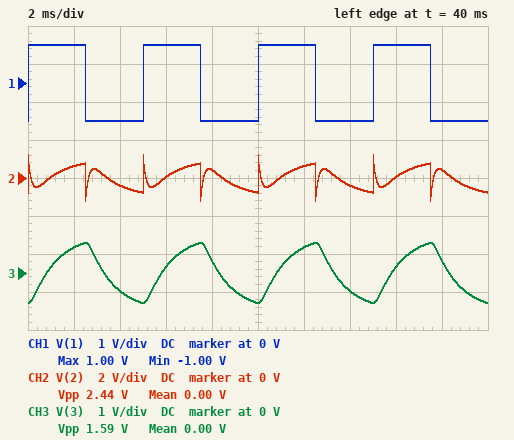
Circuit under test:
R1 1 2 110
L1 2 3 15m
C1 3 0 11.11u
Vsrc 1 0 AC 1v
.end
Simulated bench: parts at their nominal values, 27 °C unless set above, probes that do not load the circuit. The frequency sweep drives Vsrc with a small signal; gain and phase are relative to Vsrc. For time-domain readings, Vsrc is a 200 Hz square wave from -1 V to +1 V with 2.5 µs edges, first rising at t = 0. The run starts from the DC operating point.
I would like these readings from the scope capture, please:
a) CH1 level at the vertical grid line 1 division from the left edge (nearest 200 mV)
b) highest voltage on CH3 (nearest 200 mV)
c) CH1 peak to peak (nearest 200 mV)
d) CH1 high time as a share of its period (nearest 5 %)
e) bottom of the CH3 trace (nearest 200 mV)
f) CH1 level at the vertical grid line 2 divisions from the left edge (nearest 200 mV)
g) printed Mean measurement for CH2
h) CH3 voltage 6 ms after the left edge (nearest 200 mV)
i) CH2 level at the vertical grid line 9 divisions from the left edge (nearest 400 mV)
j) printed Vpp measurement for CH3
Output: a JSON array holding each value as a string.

["1.0 V", "800 mV", "2.0 V", "50 %", "-800 mV", "-1.0 V", "0.00 V", "200 mV", "400 mV", "1.59 V"]
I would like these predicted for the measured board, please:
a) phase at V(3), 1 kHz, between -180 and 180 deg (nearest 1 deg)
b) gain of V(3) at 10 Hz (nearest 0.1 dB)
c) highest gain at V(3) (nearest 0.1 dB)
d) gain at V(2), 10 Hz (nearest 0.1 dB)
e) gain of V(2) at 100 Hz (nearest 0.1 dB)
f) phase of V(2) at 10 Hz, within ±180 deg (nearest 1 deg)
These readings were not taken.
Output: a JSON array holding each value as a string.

["-126 deg", "0 dB", "0 dB", "0 dB", "-2.2 dB", "-4 deg"]
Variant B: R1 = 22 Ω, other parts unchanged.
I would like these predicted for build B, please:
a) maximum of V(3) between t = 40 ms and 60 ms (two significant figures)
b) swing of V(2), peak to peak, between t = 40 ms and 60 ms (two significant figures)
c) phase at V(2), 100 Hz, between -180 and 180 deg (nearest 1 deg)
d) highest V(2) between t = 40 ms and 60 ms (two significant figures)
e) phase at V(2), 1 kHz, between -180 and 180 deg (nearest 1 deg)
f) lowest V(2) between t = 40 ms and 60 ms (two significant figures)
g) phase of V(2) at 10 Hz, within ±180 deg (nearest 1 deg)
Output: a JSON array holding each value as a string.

["1.7 V", "2.5 V", "-9 deg", "1.3 V", "15 deg", "-1.3 V", "-1 deg"]
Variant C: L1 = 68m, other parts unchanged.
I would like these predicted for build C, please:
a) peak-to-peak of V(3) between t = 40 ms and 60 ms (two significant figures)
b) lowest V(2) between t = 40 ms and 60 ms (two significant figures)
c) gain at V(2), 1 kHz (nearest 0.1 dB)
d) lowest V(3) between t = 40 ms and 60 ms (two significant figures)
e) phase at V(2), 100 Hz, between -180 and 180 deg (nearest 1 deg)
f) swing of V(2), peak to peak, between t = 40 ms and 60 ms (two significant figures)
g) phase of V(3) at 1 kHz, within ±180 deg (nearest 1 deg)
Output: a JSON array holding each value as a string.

["1.7 V", "-1.5 V", "-0.3 dB", "-870 mV", "-48 deg", "3.0 V", "-165 deg"]
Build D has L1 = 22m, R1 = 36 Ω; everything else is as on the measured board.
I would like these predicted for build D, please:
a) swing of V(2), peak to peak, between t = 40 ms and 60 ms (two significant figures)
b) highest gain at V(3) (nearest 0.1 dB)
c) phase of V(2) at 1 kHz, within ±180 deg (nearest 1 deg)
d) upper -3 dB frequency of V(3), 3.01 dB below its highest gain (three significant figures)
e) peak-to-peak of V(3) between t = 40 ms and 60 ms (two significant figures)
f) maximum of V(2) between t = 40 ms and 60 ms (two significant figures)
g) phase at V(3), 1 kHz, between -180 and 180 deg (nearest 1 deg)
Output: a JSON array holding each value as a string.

["2.5 V", "2.6 dB", "16 deg", "383 Hz", "3.1 V", "1.3 V", "-164 deg"]
